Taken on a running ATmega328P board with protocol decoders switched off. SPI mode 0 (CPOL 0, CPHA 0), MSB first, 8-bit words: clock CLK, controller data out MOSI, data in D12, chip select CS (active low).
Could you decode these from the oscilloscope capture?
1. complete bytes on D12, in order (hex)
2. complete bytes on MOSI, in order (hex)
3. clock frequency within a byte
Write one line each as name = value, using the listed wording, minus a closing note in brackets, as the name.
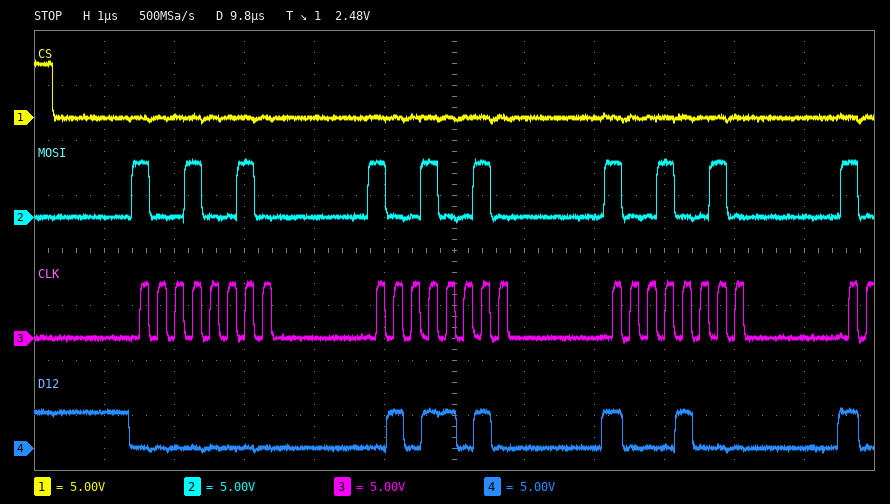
complete bytes on D12, in order = 00 5A 88
complete bytes on MOSI, in order = 92 92 92
clock frequency within a byte = 4 MHz
